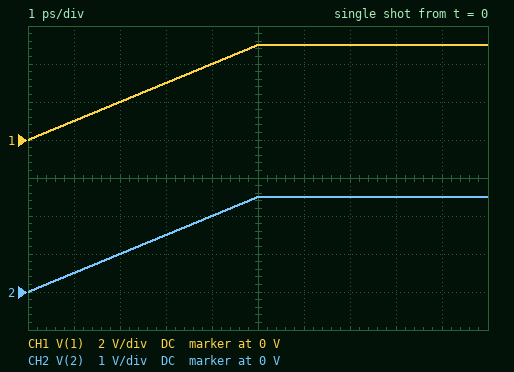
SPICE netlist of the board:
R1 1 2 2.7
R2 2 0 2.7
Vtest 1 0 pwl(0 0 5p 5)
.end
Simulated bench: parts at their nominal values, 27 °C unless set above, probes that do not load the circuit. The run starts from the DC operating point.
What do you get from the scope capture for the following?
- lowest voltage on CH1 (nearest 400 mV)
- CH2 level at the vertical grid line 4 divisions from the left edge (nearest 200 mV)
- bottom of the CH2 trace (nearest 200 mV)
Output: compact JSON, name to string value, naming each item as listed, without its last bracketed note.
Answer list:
{"lowest voltage on CH1": "0 V", "CH2 level at the vertical grid line 4 divisions from the left edge": "2.0 V", "bottom of the CH2 trace": "0 V"}
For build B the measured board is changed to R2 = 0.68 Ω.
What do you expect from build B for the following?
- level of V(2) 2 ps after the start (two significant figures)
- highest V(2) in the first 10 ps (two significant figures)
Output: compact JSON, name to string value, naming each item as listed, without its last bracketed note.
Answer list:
{"level of V(2) 2 ps after the start": "400 mV", "highest V(2) in the first 10 ps": "1.0 V"}
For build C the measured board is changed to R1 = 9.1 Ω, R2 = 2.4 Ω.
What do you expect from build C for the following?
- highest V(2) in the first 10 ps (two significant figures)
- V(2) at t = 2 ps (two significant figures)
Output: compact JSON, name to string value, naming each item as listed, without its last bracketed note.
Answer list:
{"highest V(2) in the first 10 ps": "1.0 V", "V(2) at t = 2 ps": "420 mV"}
